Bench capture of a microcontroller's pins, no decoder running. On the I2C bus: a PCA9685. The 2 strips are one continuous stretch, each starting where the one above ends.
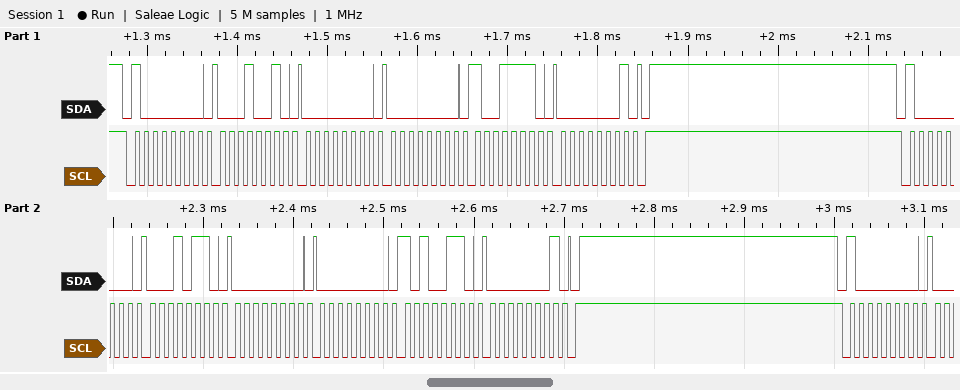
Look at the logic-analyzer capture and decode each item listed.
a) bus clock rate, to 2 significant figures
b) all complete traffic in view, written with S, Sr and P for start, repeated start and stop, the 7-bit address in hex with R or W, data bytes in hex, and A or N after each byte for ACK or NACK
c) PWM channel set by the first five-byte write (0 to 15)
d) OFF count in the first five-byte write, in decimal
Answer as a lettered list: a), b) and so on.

a) 100 kHz
b) S 40W A 12 A 00 A 00 A 9E A 01 A P S 40W A 16 A 00 A 00 A A6 A 01 A P S 40W A
c) 3
d) 414
